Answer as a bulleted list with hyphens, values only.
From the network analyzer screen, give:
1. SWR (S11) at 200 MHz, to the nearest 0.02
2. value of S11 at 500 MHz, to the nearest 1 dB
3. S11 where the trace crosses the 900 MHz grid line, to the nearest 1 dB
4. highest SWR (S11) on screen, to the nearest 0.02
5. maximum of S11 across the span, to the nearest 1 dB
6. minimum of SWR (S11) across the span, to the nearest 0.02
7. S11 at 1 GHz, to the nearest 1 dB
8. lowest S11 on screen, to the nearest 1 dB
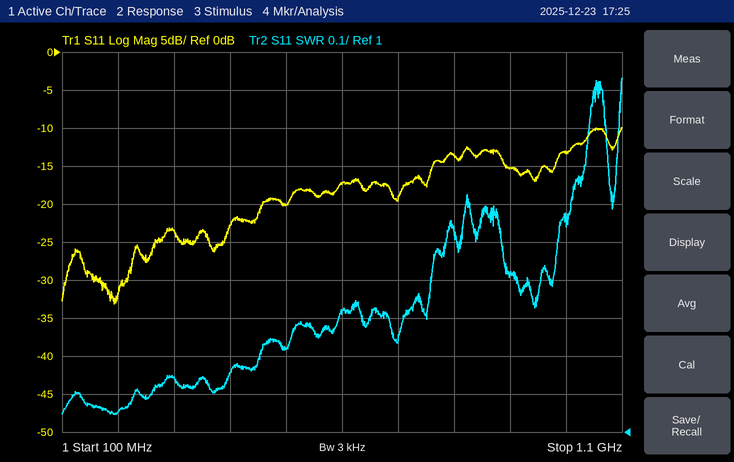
- 1.06
- -20 dB
- -15 dB
- 1.94
- -10 dB
- 1.04
- -13 dB
- -33 dB
